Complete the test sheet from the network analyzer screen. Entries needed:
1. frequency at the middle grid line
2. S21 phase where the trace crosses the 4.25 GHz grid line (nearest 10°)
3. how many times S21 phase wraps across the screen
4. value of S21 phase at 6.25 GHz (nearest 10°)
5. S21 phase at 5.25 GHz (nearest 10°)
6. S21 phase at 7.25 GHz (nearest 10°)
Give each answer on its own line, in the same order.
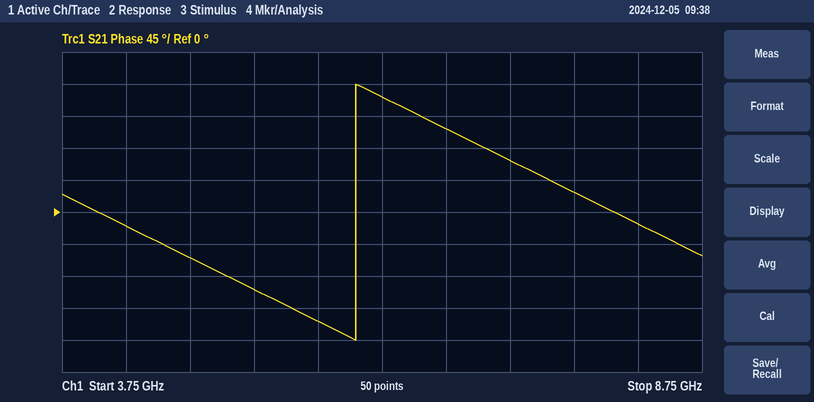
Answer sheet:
6.25 GHz
-20°
1
160°
-110°
70°
